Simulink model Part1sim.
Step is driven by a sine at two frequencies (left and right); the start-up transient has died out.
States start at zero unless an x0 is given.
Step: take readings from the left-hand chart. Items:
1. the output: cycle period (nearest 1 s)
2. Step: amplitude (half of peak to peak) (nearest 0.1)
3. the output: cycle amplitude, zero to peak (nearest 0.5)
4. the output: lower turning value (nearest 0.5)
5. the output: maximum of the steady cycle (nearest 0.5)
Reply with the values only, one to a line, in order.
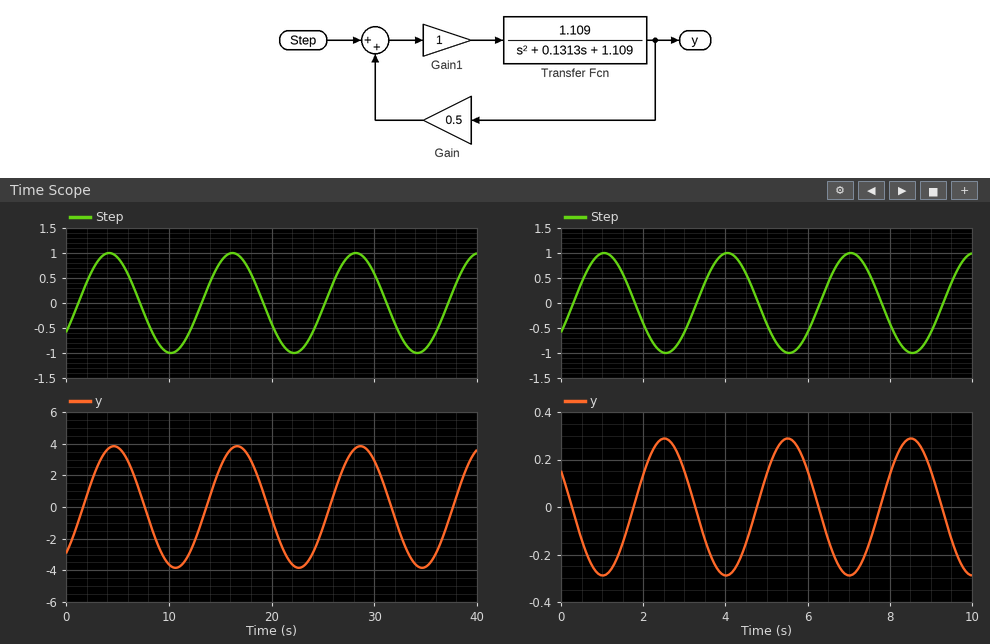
12 s
1.0
4.0
-4.0
4.0
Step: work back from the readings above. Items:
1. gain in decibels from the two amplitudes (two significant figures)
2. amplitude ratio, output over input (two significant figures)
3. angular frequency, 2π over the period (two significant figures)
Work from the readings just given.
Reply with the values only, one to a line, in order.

12 dB
4.0
0.52 rad/s
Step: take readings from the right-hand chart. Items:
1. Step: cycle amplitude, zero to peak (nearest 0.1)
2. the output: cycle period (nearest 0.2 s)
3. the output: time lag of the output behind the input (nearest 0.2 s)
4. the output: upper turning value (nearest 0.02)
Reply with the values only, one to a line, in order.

1.0
3.0 s
1.4 s
0.28
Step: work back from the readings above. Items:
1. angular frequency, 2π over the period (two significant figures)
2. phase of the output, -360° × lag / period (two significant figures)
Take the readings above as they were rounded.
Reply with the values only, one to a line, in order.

2.1 rad/s
-170°
